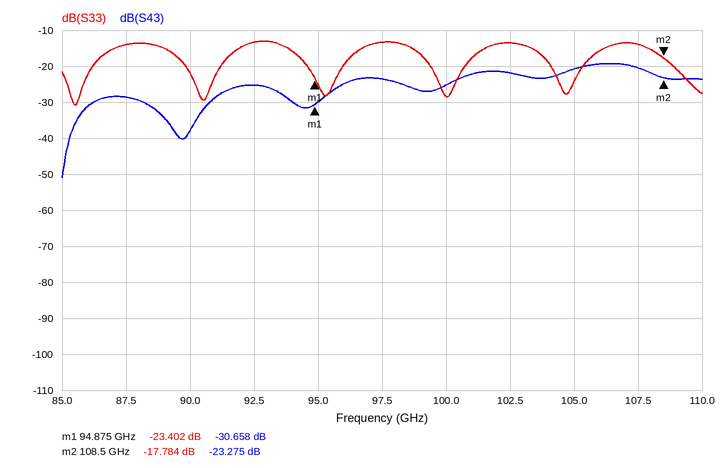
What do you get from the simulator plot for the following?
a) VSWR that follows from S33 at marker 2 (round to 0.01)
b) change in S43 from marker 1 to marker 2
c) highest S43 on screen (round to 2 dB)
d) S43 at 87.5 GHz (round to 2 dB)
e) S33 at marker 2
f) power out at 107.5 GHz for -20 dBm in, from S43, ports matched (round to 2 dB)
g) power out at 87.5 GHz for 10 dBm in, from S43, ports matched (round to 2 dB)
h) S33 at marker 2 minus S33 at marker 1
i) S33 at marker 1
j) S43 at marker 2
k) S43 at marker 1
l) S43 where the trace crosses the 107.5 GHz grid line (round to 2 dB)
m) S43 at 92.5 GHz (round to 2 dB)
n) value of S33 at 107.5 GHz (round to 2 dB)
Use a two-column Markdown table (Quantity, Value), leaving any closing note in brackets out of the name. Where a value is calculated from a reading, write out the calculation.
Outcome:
| Quantity | Value |
|---|---|
| VSWR that follows from S33 at marker 2 | (1 + 0.1291)/(1 − 0.1291) ≈ 1.30 |
| change in S43 from marker 1 to marker 2 | -23.275 − (-30.658) = 7.383 dB |
| highest S43 on screen | -20 dB |
| S43 at 87.5 GHz | -28 dB |
| S33 at marker 2 | -17.784 dB |
| power out at 107.5 GHz for -20 dBm in, from S43, ports matched | -20 dBm + (-20 dB) = -40 dBm |
| power out at 87.5 GHz for 10 dBm in, from S43, ports matched | 10 dBm + (-28 dB) = -18 dBm |
| S33 at marker 2 minus S33 at marker 1 | -17.784 − (-23.402) = 5.618 dB |
| S33 at marker 1 | -23.402 dB |
| S43 at marker 2 | -23.275 dB |
| S43 at marker 1 | -30.658 dB |
| S43 where the trace crosses the 107.5 GHz grid line | -20 dB |
| S43 at 92.5 GHz | -26 dB |
| value of S33 at 107.5 GHz | -14 dB |
